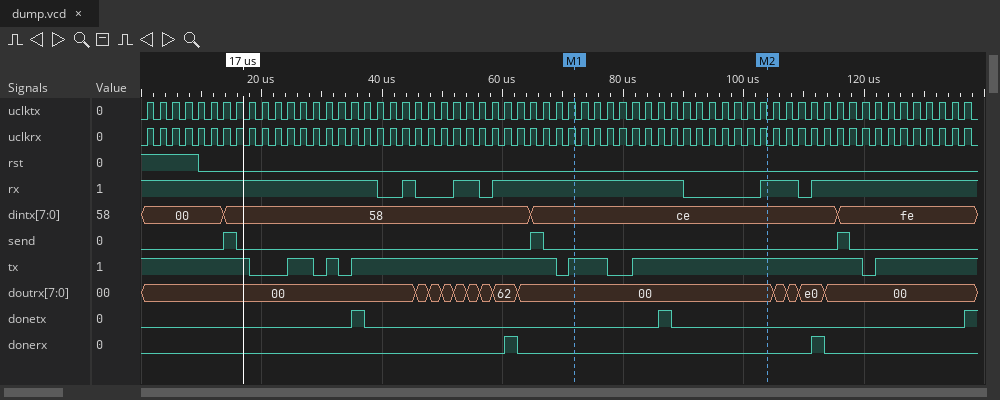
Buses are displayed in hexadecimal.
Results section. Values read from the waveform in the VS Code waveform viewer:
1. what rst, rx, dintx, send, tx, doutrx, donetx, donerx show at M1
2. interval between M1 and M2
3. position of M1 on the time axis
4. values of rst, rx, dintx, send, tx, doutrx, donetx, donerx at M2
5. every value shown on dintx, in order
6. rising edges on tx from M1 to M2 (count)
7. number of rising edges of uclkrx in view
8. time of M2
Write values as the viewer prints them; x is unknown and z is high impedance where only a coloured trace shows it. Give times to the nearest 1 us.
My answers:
rst=0, rx=1, dintx=ce, send=0, tx=1, doutrx=00, donetx=0, donerx=0
32 us
72 us
rst=0, rx=1, dintx=ce, send=0, tx=1, doutrx=00, donetx=0, donerx=0
00, 58, ce, fe
1
65
104 us
